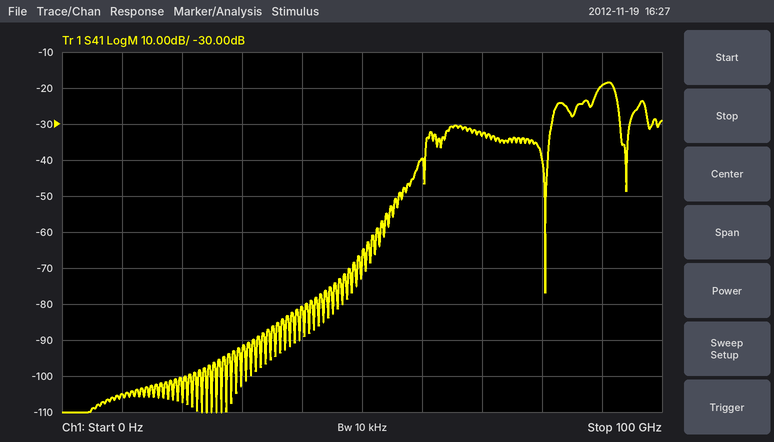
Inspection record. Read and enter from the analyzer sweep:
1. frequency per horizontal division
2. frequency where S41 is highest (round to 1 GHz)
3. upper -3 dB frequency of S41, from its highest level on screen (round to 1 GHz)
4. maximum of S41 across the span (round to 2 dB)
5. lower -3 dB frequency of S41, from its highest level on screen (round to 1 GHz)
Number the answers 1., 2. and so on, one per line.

1. 10 GHz
2. 91 GHz
3. 92 GHz
4. -18 dB
5. 89 GHz
